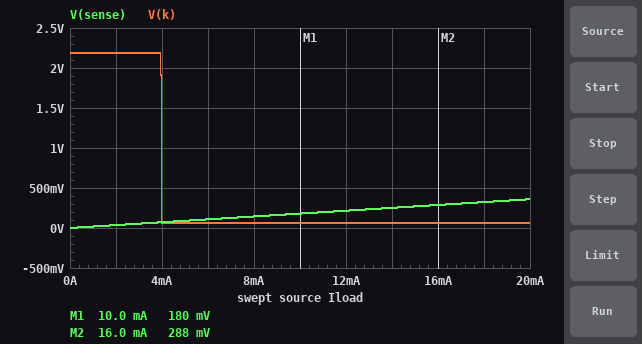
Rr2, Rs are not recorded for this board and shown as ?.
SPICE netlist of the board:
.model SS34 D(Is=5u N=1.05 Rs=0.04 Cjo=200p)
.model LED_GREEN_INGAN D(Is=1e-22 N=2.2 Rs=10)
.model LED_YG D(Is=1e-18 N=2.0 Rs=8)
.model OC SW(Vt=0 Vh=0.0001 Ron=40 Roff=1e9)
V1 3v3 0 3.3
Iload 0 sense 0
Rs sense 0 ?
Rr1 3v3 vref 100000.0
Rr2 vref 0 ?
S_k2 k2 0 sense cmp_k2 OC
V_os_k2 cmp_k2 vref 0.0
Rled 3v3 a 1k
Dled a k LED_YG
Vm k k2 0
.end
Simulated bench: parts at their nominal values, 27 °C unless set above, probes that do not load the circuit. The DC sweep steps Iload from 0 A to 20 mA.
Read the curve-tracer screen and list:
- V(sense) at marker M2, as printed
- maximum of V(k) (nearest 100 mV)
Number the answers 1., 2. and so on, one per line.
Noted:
1. 288 mV
2. 2.2 V
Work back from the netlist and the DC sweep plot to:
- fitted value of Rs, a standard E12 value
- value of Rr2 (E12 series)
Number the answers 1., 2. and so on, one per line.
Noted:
1. 18 Ω
2. 2.2 kΩ
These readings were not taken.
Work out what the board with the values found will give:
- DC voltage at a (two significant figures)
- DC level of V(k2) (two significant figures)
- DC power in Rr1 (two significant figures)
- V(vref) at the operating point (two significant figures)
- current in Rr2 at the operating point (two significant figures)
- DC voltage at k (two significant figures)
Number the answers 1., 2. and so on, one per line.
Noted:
1. 3.3 V
2. 2.2 V
3. 100 µW
4. 71 mV
5. 32 µA
6. 2.2 V
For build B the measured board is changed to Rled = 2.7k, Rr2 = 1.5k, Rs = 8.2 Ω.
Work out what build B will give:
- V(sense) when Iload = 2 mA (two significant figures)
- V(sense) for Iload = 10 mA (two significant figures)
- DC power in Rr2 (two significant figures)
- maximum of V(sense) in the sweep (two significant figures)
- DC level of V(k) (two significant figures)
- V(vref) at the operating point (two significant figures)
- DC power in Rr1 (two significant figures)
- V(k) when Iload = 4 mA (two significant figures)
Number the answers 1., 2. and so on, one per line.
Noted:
1. 16 mV
2. 82 mV
3. 1.6 µW
4. 160 mV
5. 2.2 V
6. 49 mV
7. 110 µW
8. 2.2 V
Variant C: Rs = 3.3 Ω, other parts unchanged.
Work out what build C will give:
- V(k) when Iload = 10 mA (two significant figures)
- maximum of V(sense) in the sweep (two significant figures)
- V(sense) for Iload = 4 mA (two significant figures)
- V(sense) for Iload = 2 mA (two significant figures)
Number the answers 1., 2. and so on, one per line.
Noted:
1. 2.2 V
2. 66 mV
3. 13 mV
4. 6.6 mV
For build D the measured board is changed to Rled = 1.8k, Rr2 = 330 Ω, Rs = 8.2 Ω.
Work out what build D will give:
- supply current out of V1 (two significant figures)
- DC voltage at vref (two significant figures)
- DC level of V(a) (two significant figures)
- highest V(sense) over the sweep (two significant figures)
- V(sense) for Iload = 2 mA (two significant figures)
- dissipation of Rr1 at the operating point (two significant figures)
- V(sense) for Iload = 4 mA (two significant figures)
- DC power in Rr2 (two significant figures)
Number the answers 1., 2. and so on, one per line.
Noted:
1. 33 µA
2. 11 mV
3. 3.3 V
4. 160 mV
5. 16 mV
6. 110 µW
7. 33 mV
8. 360 nW
